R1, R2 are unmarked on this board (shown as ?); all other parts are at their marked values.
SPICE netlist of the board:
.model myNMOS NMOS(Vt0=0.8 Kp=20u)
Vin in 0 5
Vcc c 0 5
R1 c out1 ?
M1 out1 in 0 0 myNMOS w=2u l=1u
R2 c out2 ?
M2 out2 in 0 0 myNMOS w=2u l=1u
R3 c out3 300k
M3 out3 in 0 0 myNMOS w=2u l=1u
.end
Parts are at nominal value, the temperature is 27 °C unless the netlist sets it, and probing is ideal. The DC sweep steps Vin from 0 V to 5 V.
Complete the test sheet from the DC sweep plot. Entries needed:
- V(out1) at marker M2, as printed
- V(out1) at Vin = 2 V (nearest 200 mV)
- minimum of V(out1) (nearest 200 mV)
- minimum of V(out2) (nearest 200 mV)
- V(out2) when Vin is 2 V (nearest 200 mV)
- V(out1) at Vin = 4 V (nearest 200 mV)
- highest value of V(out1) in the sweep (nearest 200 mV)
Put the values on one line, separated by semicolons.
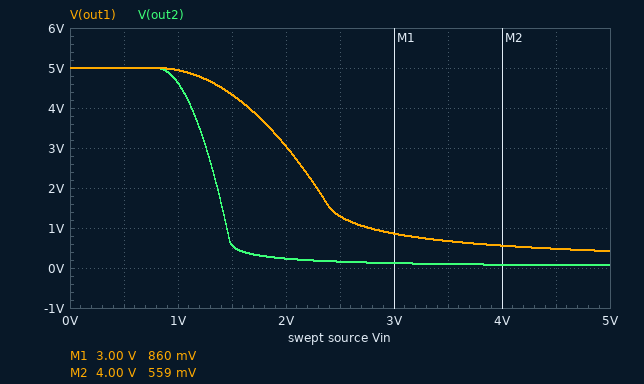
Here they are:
559 mV; 3.0 V; 400 mV; 0 V; 200 mV; 600 mV; 5.0 V
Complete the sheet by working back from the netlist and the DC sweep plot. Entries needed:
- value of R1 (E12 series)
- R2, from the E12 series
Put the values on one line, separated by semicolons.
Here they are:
68 kΩ; 470 kΩ
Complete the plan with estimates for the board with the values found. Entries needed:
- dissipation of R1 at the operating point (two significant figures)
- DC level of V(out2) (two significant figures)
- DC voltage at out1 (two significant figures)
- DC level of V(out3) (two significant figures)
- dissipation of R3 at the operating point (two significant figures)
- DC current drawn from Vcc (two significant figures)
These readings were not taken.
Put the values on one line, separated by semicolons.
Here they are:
310 µW; 63 mV; 420 mV; 98 mV; 80 µW; 94 µA
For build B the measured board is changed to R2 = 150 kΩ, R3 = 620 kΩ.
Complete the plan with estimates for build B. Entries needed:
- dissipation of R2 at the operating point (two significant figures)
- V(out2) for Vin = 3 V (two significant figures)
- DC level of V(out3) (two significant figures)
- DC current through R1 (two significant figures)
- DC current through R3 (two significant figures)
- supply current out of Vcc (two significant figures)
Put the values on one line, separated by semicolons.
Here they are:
150 µW; 380 mV; 48 mV; 67 µA; 8.0 µA; 110 µA
